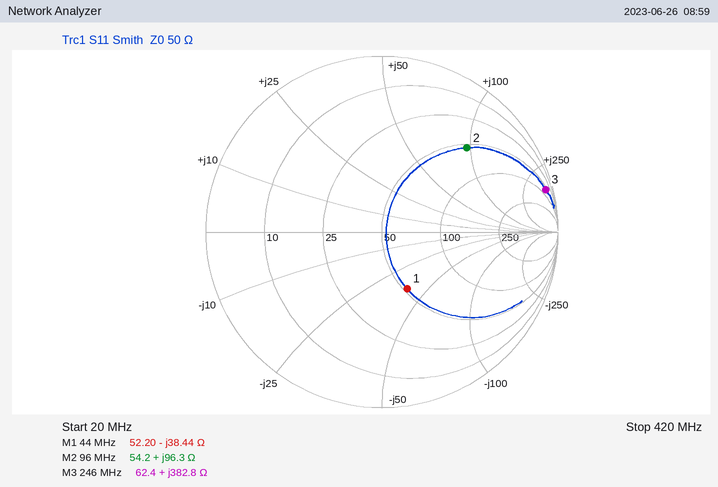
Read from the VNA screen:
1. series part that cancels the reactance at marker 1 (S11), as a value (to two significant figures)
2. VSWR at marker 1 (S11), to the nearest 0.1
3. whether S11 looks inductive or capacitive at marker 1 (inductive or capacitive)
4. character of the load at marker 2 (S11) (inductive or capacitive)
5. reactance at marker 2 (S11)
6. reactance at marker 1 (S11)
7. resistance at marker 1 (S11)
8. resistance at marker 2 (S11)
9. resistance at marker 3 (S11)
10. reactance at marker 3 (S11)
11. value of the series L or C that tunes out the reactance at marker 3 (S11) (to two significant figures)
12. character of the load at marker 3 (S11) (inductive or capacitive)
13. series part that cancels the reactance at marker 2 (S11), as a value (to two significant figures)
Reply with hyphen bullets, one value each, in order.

- 140 nH
- 2.1
- capacitive
- inductive
- +96.3 Ω
- -38.44 Ω
- 52.20 Ω
- 54.2 Ω
- 62.4 Ω
- +382.8 Ω
- 1.7 pF
- inductive
- 17 pF
